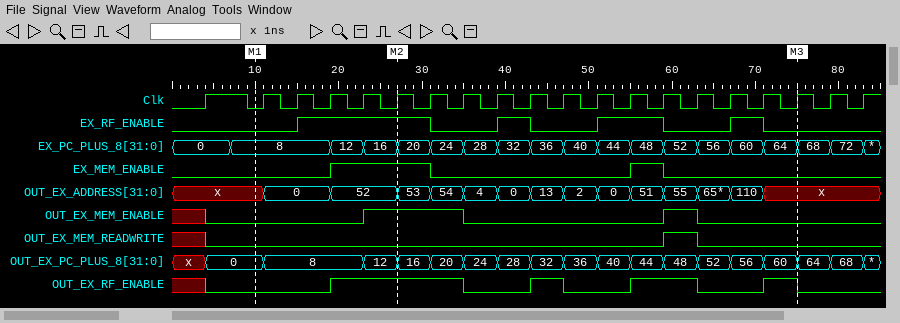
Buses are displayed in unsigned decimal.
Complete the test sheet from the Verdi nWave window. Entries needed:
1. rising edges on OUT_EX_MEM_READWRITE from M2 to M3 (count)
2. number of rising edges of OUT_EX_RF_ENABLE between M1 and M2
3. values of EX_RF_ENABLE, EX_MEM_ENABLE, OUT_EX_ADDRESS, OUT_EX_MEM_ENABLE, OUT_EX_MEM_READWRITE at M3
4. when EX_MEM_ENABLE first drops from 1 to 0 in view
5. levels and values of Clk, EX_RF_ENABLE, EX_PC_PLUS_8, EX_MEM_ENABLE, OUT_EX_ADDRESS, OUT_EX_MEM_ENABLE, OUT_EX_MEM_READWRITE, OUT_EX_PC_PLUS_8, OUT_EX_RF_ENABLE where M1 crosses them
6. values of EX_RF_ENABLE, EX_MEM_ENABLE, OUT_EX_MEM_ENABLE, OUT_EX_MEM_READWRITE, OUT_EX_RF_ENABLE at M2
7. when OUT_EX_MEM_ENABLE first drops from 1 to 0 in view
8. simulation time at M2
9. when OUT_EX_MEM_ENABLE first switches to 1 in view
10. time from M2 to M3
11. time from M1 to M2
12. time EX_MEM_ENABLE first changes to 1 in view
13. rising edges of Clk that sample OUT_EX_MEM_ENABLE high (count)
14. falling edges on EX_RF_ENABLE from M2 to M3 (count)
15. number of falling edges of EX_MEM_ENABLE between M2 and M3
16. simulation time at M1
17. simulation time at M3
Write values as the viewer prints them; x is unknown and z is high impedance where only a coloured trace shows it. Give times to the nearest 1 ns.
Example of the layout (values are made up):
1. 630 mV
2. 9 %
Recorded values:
1. 1
2. 1
3. EX_RF_ENABLE=0, EX_MEM_ENABLE=0, OUT_EX_ADDRESS=x, OUT_EX_MEM_ENABLE=0, OUT_EX_MEM_READWRITE=0
4. 31 ns
5. Clk=0, EX_RF_ENABLE=0, EX_PC_PLUS_8=8, EX_MEM_ENABLE=0, OUT_EX_ADDRESS=x, OUT_EX_MEM_ENABLE=0, OUT_EX_MEM_READWRITE=0, OUT_EX_PC_PLUS_8=0, OUT_EX_RF_ENABLE=0
6. EX_RF_ENABLE=1, EX_MEM_ENABLE=1, OUT_EX_MEM_ENABLE=1, OUT_EX_MEM_READWRITE=0, OUT_EX_RF_ENABLE=1
7. 35 ns
8. 27 ns
9. 23 ns
10. 48 ns
11. 17 ns
12. 19 ns
13. 4
14. 4
15. 2
16. 10 ns
17. 75 ns
